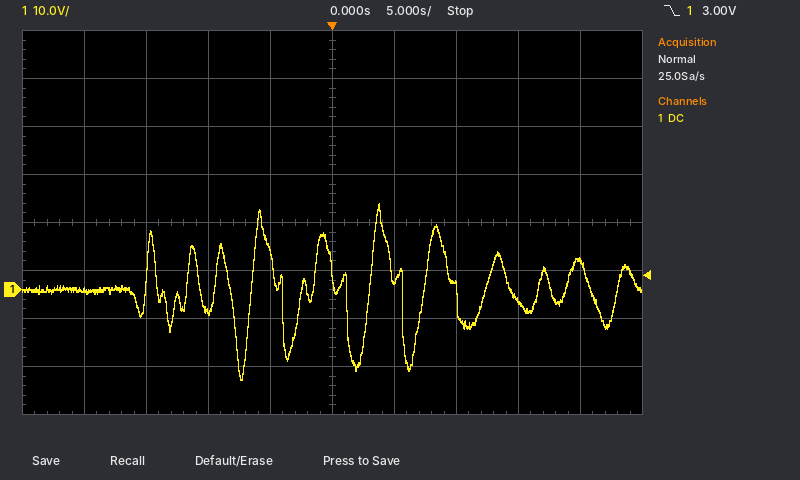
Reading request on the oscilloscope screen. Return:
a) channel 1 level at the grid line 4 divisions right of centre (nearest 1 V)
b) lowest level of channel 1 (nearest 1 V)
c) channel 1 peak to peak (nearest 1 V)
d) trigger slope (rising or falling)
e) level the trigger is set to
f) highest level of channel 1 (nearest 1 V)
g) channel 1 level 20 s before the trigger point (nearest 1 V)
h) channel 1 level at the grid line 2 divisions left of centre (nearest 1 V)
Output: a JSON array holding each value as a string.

["6 V", "-19 V", "37 V", "falling", "3.00 V", "18 V", "0 V", "-4 V"]
